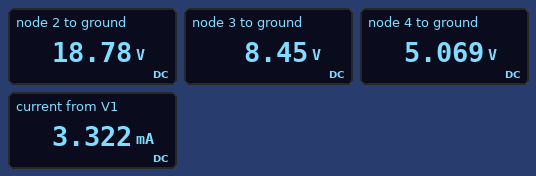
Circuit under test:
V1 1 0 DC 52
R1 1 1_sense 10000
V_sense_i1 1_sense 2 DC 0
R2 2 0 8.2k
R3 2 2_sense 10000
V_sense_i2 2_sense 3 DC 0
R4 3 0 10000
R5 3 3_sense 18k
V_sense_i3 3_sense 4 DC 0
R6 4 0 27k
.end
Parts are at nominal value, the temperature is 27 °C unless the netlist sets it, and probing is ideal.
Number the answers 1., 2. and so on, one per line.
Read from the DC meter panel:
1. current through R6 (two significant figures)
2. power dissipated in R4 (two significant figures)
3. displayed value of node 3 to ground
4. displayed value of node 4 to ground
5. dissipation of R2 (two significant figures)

1. 190 µA
2. 7.1 mW
3. 8.45 V
4. 5.069 V
5. 43 mW
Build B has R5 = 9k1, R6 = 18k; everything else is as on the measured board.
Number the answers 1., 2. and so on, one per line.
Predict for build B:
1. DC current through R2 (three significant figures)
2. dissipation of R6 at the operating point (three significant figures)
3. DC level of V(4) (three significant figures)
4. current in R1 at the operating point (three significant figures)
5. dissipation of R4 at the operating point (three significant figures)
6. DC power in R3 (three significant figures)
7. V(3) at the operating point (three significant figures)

1. 2.27 mA
2. 1.51 mW
3. 5.21 V
4. 3.34 mA
5. 6.16 mW
6. 11.5 mW
7. 7.85 V
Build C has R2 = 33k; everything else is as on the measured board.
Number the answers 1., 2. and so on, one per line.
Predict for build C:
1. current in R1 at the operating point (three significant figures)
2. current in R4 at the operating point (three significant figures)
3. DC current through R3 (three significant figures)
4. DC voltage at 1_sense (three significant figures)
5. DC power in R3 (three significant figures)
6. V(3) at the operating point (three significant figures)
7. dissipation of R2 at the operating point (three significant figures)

1. 2.39 mA
2. 1.26 mA
3. 1.54 mA
4. 28.1 V
5. 23.8 mW
6. 12.6 V
7. 23.9 mW
